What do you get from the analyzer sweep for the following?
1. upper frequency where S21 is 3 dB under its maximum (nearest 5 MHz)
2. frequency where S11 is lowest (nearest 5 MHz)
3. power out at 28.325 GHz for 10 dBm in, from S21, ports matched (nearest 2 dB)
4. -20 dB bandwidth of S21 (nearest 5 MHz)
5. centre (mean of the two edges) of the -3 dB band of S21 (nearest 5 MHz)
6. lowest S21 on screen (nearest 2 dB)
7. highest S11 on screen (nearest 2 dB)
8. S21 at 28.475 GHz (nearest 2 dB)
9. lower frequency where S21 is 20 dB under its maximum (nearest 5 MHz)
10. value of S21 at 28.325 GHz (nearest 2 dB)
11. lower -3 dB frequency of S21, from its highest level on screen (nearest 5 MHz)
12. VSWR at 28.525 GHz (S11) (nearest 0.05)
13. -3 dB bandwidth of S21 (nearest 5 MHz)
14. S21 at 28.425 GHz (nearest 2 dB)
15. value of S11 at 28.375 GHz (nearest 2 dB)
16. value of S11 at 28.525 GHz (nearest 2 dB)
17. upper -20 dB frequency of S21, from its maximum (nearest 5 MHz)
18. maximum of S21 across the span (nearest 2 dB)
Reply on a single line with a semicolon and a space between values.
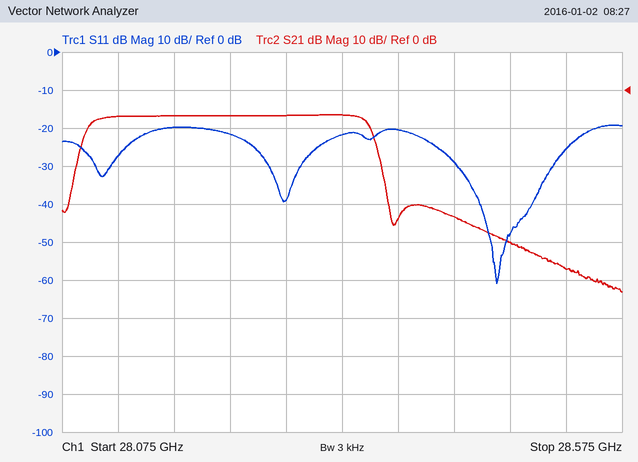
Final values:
28.350 GHz; 28.465 GHz; 4 dBm; 280 MHz; 28.225 GHz; -54 dB; -20 dB; -40 dB; 28.085 GHz; -6 dB; 28.100 GHz; 1.10; 250 MHz; -34 dB; -20 dB; -26 dB; 28.365 GHz; -6 dB
